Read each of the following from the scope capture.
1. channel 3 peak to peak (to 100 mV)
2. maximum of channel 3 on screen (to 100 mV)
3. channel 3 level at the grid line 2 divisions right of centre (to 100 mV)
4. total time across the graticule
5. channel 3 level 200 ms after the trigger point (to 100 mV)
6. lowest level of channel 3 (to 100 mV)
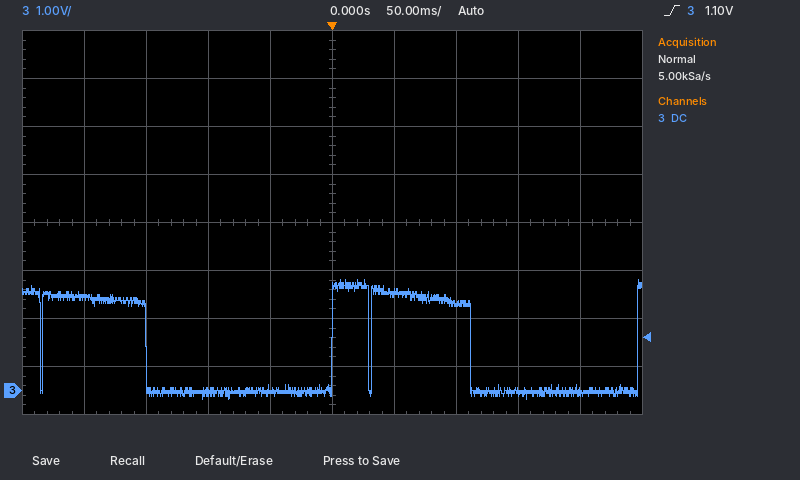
2.5 V
2.3 V
1.8 V
500 ms
0.0 V
-200 mV
